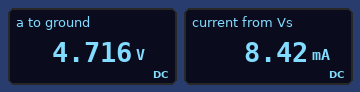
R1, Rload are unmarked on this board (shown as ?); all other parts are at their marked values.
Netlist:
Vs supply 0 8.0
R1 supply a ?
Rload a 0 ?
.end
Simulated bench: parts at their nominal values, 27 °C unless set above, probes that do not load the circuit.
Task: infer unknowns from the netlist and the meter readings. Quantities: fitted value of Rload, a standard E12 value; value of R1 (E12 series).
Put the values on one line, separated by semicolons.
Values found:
560 Ω; 390 Ω
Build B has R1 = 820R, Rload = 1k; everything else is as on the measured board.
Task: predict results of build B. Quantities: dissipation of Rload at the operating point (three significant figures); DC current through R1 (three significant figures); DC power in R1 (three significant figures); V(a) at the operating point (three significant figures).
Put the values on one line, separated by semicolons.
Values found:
19.3 mW; 4.40 mA; 15.8 mW; 4.40 V
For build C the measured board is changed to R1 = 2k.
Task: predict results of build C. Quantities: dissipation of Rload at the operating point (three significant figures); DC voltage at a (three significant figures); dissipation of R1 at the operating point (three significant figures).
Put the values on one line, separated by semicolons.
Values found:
5.47 mW; 1.75 V; 19.5 mW
